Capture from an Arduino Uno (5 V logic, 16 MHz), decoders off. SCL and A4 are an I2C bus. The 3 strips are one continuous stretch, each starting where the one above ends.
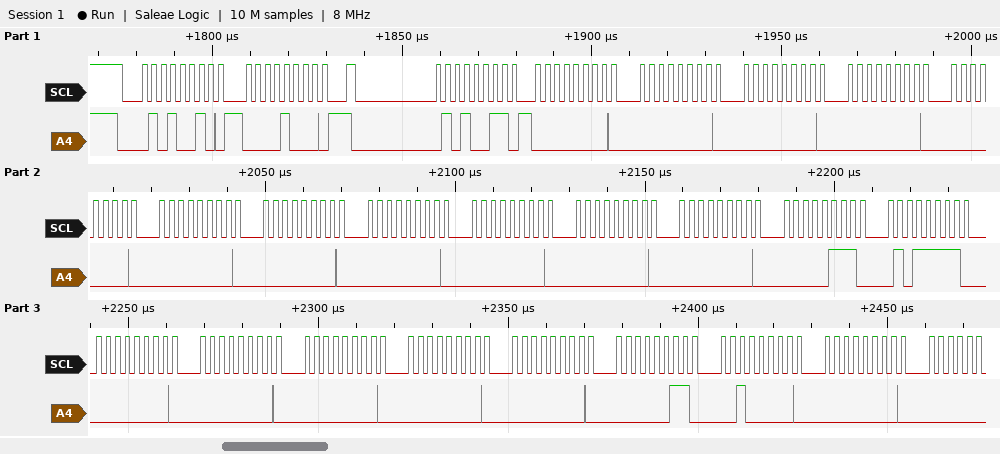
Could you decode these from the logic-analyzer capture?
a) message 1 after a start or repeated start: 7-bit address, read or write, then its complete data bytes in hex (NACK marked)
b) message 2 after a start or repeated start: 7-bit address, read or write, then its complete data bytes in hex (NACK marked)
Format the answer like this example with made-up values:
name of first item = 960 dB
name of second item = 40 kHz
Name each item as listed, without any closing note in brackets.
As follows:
message 1 after a start or repeated start: 7-bit address, read or write, then its complete data bytes in hex = 0x29 write: 08
message 2 after a start or repeated start: 7-bit address, read or write, then its complete data bytes in hex = 0x29 read: 00 00 00 00 00 00 00 00 00 00 00 07 5F 00 00 00 00 00 03 20 00
